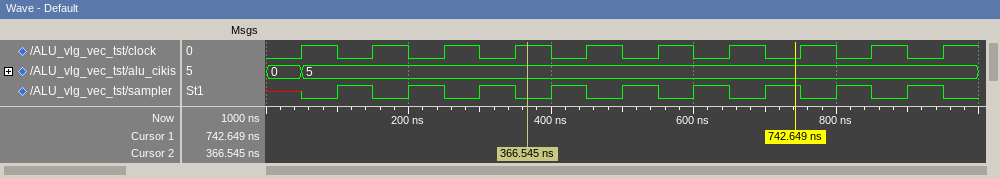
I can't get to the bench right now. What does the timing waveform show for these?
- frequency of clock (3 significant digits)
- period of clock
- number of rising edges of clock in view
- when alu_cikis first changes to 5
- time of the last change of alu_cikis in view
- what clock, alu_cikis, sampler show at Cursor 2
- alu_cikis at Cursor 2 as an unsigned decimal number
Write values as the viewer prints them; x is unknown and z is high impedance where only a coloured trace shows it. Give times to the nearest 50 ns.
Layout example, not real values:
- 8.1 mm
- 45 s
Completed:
- 10.0 MHz
- 100 ns
- 10
- 50 ns
- 50 ns
- clock=1, alu_cikis=5, sampler=0
- 5
